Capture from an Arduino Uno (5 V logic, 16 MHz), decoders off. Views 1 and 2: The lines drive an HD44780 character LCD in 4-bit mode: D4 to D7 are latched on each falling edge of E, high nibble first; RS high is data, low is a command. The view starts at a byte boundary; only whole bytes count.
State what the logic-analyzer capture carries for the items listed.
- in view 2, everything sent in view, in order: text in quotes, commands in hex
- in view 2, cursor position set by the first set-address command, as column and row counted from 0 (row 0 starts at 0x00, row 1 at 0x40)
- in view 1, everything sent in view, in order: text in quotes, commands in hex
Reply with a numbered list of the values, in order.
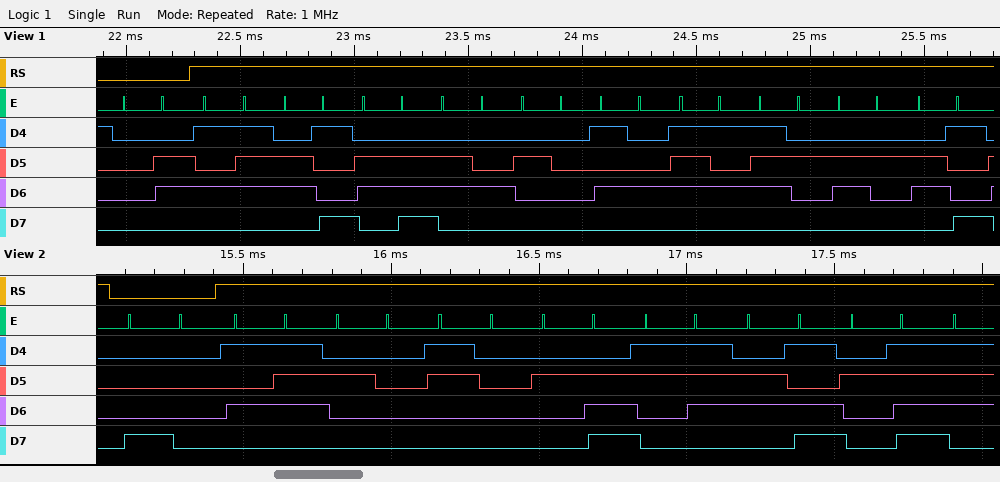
1. 0x80 "W 0.7m/"
2. column 0, row 0
3. 0x06 "Wind Turbi"
